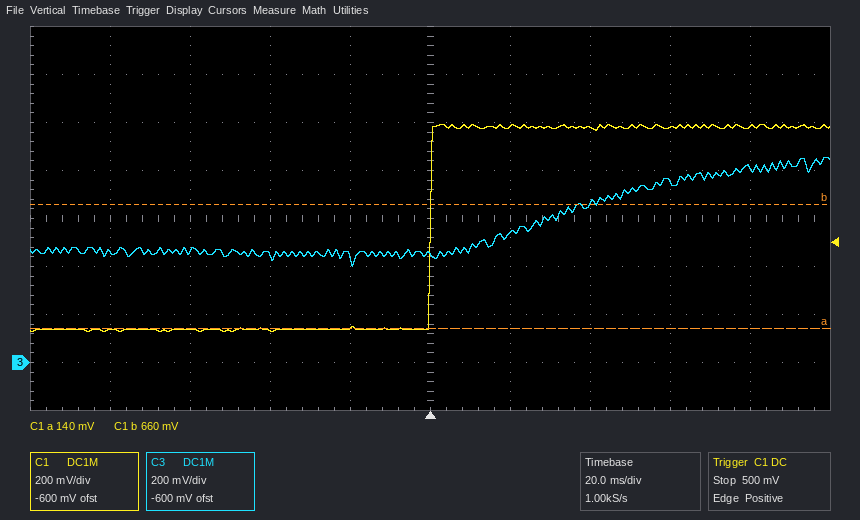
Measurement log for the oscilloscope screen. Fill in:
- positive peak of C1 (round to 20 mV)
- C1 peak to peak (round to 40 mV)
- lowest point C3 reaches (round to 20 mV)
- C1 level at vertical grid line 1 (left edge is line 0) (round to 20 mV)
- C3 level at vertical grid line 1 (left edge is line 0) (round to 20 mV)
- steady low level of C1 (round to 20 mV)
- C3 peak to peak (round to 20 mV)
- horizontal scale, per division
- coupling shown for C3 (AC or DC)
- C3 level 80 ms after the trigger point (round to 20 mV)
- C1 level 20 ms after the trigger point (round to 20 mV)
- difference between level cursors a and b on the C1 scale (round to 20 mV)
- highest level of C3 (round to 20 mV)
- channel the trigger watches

1.00 V
880 mV
400 mV
140 mV
460 mV
140 mV
460 mV
20 ms
DC
800 mV
980 mV
520 mV
860 mV
C1
